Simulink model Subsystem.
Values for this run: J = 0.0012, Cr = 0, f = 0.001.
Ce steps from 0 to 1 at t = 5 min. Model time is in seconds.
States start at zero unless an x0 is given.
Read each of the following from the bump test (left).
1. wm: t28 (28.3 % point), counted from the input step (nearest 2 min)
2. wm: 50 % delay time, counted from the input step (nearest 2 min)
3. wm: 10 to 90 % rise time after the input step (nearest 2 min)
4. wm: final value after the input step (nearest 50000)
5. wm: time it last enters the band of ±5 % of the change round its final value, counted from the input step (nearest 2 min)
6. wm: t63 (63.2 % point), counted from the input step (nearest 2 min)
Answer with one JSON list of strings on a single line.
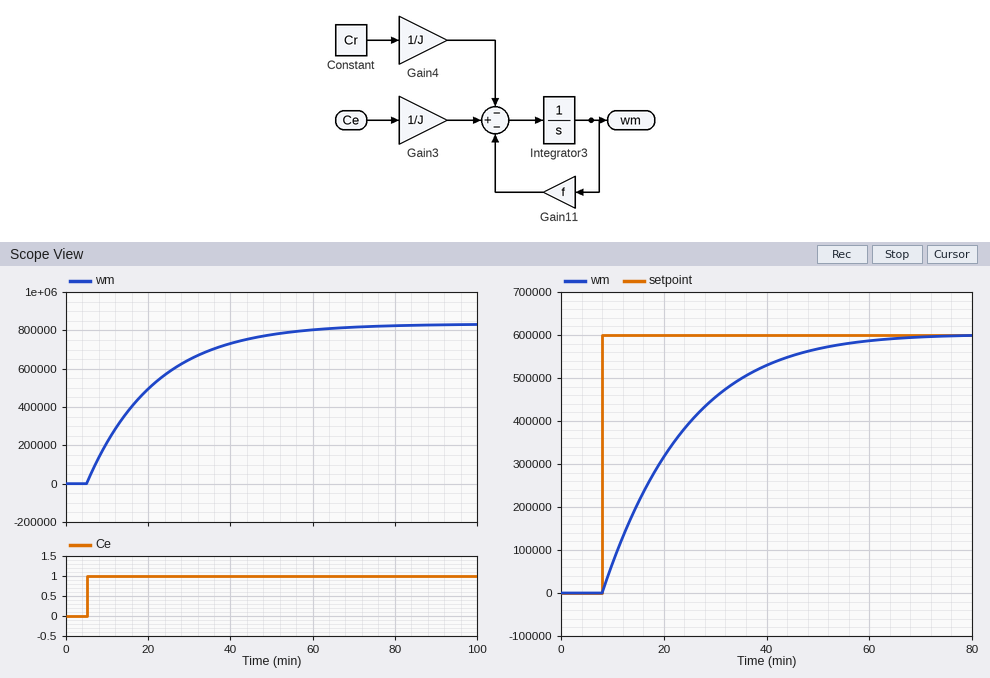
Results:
["6 min", "12 min", "36 min", "850000", "50 min", "16 min"]
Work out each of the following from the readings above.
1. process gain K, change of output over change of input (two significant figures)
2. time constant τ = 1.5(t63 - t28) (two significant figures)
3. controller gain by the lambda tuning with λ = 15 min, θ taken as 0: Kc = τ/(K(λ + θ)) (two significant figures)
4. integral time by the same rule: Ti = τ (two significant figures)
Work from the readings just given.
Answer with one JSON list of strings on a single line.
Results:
["850000", "15 min", "0.0000012", "15 min"]
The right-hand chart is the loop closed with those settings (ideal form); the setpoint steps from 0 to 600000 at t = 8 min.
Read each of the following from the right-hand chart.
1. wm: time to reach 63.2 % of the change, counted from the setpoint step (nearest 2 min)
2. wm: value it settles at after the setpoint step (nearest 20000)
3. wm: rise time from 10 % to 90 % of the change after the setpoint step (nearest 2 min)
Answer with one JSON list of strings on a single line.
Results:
["16 min", "600000", "32 min"]
